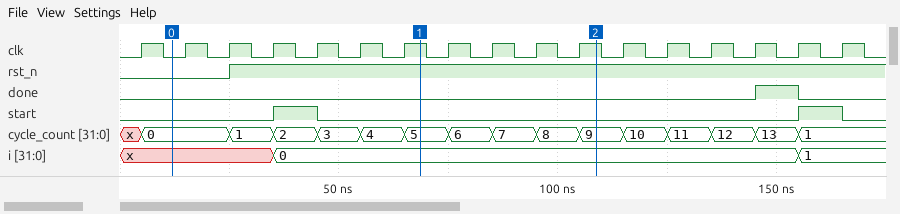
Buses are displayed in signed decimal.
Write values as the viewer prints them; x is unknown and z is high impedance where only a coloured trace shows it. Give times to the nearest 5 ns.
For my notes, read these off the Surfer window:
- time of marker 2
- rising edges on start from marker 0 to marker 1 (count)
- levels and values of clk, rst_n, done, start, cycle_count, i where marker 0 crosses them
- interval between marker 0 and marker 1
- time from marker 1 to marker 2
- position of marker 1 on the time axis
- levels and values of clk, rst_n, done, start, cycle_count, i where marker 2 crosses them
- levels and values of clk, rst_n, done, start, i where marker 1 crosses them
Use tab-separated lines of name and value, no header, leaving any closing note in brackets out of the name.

time of marker 2	110 ns
rising edges on start from marker 0 to marker 1	1
levels and values of clk, rst_n, done, start, cycle_count, i where marker 0 crosses them	clk=0, rst_n=0, done=0, start=0, cycle_count=0, i=x
interval between marker 0 and marker 1	55 ns
time from marker 1 to marker 2	40 ns
position of marker 1 on the time axis	70 ns
levels and values of clk, rst_n, done, start, cycle_count, i where marker 2 crosses them	clk=1, rst_n=1, done=0, start=0, cycle_count=9, i=0
levels and values of clk, rst_n, done, start, i where marker 1 crosses them	clk=1, rst_n=1, done=0, start=0, i=0
